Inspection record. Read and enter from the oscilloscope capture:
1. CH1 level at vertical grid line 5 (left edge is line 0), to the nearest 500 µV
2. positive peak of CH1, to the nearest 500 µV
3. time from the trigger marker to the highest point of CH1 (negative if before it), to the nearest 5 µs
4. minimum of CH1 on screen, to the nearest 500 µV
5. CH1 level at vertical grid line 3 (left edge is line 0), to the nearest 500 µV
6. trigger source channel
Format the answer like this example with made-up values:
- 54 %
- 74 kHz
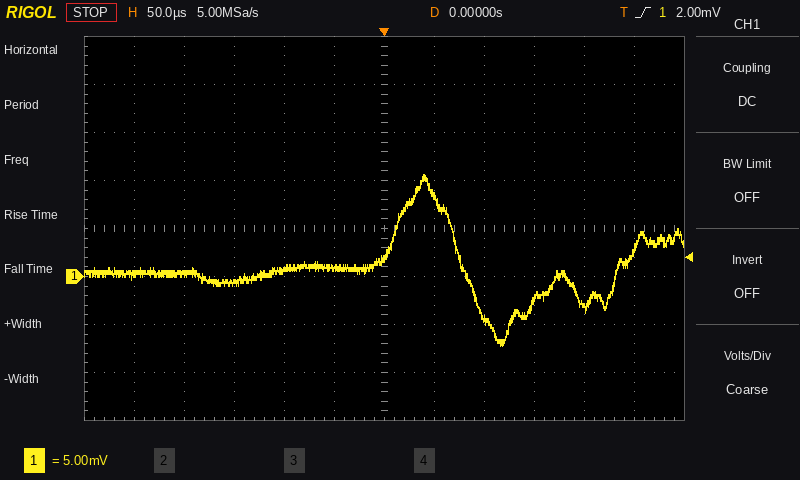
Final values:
- 1.0 mV
- 10.5 mV
- +40 µs
- -7.0 mV
- -500 µV
- CH1
